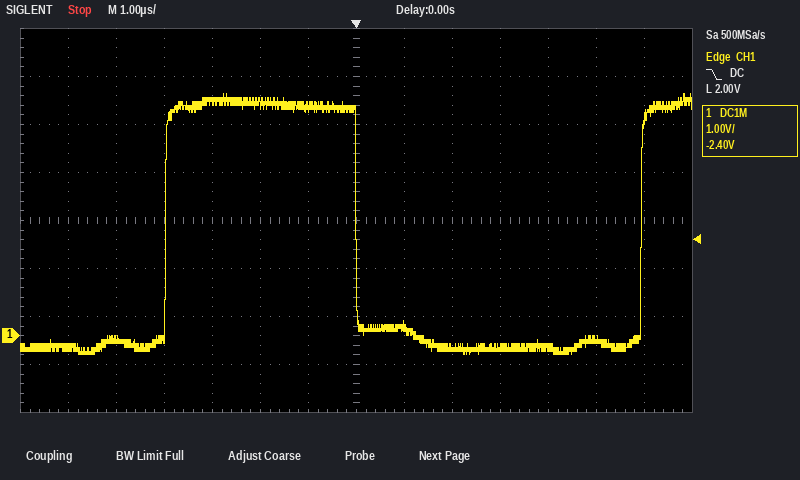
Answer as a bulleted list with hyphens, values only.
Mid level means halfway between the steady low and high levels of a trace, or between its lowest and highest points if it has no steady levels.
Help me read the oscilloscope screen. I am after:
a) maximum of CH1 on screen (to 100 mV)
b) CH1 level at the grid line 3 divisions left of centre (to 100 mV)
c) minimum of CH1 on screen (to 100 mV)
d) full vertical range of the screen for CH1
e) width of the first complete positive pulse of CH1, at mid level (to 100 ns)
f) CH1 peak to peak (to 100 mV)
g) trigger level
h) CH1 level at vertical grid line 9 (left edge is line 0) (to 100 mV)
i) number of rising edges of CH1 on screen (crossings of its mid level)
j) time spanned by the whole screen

- 5.0 V
- 4.9 V
- -400 mV
- 8 V
- 4.0 µs
- 5.4 V
- 2.00 V
- -200 mV
- 2
- 14 µs
